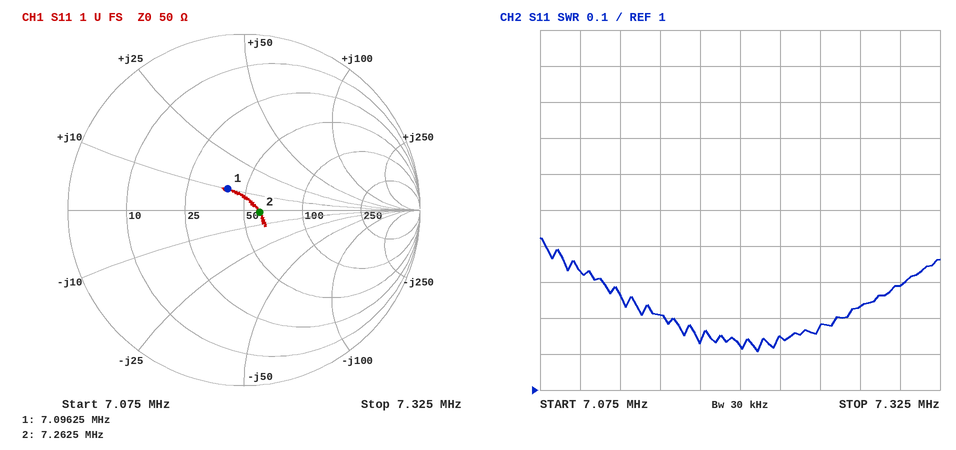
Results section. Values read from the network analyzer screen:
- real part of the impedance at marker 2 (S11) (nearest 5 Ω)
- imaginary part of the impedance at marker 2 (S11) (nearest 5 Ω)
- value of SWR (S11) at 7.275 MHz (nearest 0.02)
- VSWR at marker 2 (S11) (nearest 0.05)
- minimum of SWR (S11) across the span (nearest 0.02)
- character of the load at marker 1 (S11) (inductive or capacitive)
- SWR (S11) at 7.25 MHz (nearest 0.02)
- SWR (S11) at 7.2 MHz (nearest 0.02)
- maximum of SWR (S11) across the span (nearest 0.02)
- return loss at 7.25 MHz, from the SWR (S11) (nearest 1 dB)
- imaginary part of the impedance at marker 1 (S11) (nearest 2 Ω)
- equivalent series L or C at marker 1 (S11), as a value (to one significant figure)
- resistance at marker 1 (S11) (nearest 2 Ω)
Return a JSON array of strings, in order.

["60 Ω", "0 Ω", "1.24", "1.20", "1.10", "inductive", "1.18", "1.12", "1.42", "22 dB", "+10 Ω", "200 nH", "40 Ω"]
